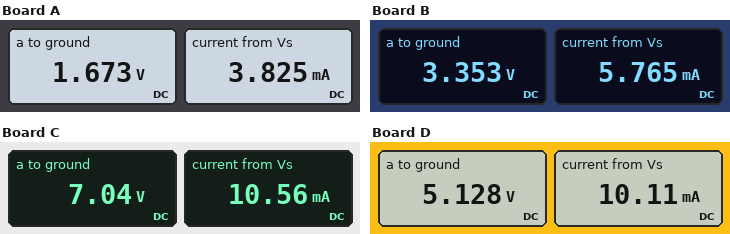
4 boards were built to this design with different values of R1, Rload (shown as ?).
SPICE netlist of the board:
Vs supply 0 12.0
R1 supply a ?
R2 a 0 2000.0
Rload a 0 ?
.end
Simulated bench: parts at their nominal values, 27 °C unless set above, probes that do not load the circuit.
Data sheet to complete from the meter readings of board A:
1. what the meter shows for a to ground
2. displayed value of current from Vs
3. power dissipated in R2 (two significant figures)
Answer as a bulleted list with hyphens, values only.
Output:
- 1.673 V
- 3.825 mA
- 1.4 mW
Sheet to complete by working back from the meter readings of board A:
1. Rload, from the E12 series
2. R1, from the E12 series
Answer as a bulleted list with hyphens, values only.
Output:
- 560 Ω
- 2.7 kΩ
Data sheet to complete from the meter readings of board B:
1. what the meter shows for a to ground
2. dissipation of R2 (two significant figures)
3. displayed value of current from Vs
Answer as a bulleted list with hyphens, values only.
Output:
- 3.353 V
- 5.6 mW
- 5.765 mA
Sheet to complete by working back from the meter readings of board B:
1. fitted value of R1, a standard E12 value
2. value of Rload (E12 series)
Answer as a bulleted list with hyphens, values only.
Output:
- 1.5 kΩ
- 820 Ω
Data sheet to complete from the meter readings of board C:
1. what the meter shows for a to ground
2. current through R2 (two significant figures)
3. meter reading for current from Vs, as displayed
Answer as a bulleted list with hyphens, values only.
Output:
- 7.04 V
- 3.5 mA
- 10.56 mA
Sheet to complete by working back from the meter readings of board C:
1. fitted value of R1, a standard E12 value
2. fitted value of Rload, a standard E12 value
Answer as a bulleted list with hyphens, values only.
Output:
- 470 Ω
- 1 kΩ
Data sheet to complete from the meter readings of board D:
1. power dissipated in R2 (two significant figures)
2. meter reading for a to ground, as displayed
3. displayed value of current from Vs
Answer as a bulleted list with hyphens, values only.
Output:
- 13 mW
- 5.128 V
- 10.11 mA
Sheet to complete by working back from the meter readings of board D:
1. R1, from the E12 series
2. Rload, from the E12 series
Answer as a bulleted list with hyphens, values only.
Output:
- 680 Ω
- 680 Ω
